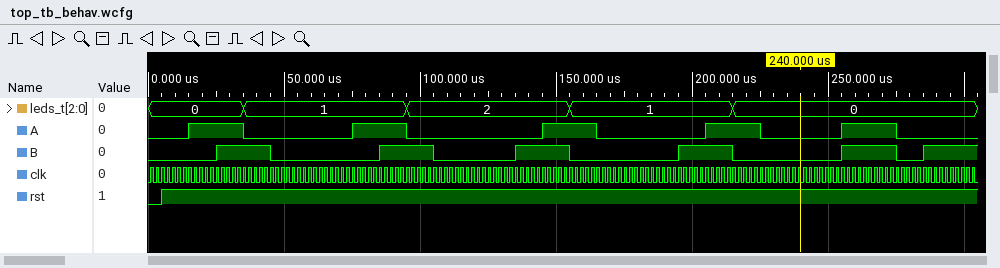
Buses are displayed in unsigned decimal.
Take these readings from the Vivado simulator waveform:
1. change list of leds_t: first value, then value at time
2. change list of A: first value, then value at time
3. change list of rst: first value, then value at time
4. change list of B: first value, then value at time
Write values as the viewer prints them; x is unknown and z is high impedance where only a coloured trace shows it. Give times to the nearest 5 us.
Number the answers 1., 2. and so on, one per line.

1. 0, 1 at 35 us, 2 at 95 us, 1 at 155 us, 0 at 215 us
2. 0, 1 at 15 us, 0 at 35 us, 1 at 75 us, 0 at 95 us, 1 at 145 us, 0 at 165 us, 1 at 205 us, 0 at 225 us, 1 at 255 us, 0 at 275 us
3. 0, 1 at 5 us
4. 0, 1 at 25 us, 0 at 45 us, 1 at 85 us, 0 at 105 us, 1 at 135 us, 0 at 155 us, 1 at 195 us, 0 at 215 us, 1 at 255 us, 0 at 275 us, 1 at 285 us
